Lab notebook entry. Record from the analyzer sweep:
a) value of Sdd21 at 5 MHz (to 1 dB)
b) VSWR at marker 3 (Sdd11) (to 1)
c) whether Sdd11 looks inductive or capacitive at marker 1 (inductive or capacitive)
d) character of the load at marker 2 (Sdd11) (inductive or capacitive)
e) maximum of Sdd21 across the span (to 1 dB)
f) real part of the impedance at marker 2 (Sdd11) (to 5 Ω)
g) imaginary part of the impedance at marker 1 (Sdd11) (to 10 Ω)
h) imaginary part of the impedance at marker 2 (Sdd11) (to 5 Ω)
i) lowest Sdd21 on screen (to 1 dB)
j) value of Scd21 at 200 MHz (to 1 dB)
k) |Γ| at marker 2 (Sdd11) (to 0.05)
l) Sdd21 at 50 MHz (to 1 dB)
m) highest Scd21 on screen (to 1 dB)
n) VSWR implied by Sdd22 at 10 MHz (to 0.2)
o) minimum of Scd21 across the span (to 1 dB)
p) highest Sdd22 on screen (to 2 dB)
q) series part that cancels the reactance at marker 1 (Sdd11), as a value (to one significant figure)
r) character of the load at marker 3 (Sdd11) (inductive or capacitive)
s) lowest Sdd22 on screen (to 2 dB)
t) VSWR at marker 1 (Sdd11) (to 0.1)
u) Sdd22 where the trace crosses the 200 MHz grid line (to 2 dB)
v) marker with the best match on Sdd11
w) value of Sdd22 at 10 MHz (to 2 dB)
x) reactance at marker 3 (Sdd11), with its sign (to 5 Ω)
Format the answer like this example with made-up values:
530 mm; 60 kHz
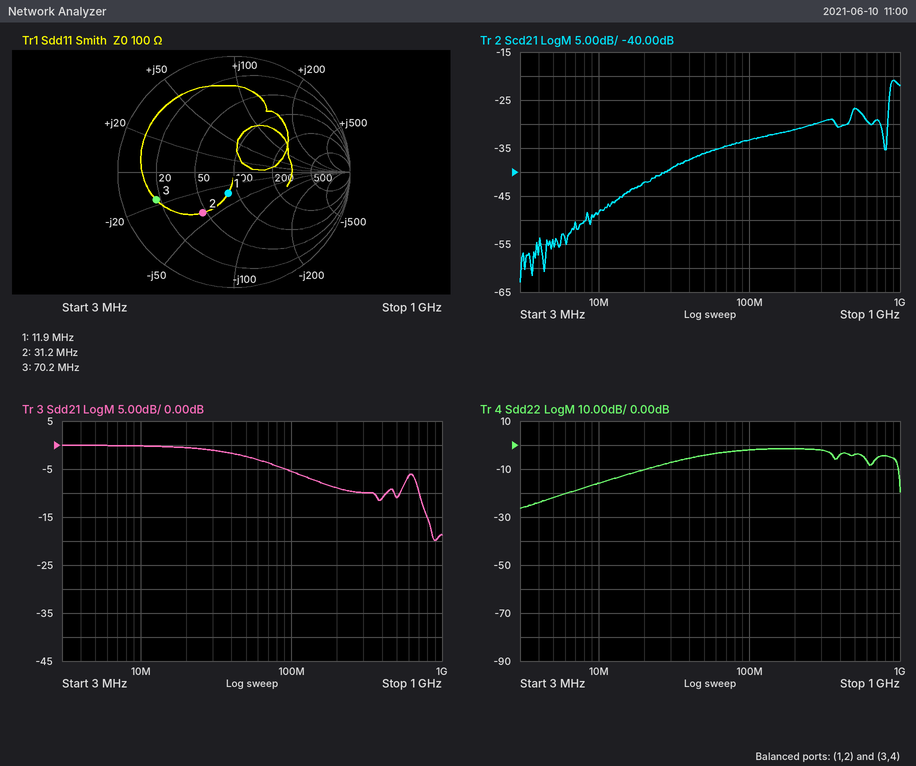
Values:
0 dB; 6; capacitive; capacitive; 0 dB; 45 Ω; -30 Ω; -40 Ω; -20 dB; -31 dB; 0.45; -2 dB; -21 dB; 1.4; -63 dB; -2 dB; 400 nH; capacitive; -26 dB; 1.5; -2 dB; marker 1; -16 dB; -15 Ω
